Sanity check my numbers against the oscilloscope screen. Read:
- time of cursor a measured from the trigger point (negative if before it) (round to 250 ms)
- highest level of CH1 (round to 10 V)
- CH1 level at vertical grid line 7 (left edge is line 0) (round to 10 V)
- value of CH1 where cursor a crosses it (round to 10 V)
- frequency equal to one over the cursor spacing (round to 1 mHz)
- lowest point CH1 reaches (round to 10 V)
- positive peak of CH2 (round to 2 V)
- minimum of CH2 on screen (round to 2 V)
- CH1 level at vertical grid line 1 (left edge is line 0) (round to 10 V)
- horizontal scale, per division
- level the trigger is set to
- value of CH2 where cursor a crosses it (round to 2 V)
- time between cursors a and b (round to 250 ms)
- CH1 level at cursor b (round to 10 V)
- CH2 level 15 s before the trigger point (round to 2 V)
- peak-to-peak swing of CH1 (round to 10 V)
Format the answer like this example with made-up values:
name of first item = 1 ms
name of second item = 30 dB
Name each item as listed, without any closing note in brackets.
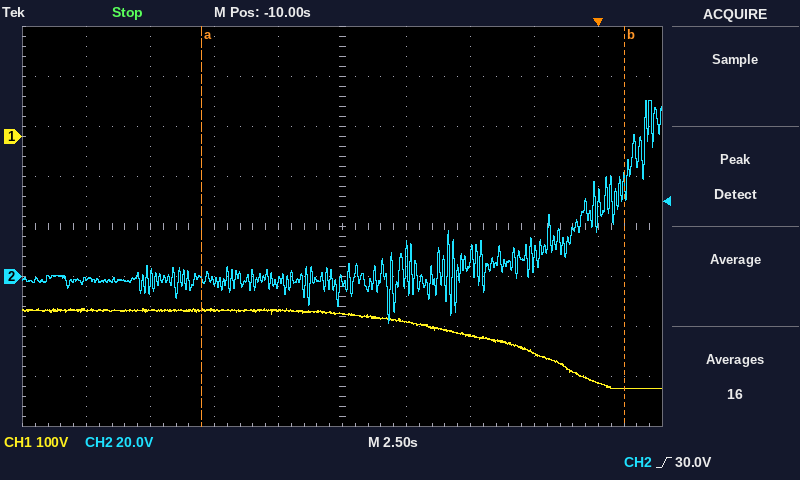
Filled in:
time of cursor a measured from the trigger point (negative if before it) = -15.50 s
highest level of CH1 = -340 V
CH1 level at vertical grid line 7 (left edge is line 0) = -400 V
value of CH1 where cursor a crosses it = -350 V
frequency equal to one over the cursor spacing = 61 mHz
lowest point CH1 reaches = -500 V
positive peak of CH2 = 70 V
minimum of CH2 on screen = -18 V
CH1 level at vertical grid line 1 (left edge is line 0) = -350 V
horizontal scale, per division = 2.5 s
level the trigger is set to = 30.0 V
value of CH2 where cursor a crosses it = -2 V
time between cursors a and b = 16.50 s
CH1 level at cursor b = -500 V
CH2 level 15 s before the trigger point = -2 V
peak-to-peak swing of CH1 = 160 V
